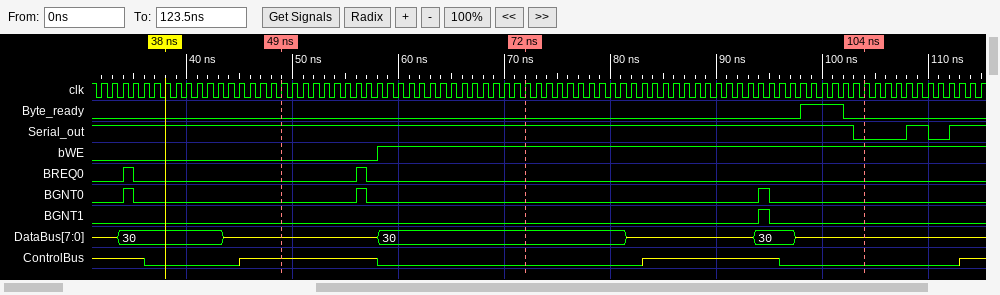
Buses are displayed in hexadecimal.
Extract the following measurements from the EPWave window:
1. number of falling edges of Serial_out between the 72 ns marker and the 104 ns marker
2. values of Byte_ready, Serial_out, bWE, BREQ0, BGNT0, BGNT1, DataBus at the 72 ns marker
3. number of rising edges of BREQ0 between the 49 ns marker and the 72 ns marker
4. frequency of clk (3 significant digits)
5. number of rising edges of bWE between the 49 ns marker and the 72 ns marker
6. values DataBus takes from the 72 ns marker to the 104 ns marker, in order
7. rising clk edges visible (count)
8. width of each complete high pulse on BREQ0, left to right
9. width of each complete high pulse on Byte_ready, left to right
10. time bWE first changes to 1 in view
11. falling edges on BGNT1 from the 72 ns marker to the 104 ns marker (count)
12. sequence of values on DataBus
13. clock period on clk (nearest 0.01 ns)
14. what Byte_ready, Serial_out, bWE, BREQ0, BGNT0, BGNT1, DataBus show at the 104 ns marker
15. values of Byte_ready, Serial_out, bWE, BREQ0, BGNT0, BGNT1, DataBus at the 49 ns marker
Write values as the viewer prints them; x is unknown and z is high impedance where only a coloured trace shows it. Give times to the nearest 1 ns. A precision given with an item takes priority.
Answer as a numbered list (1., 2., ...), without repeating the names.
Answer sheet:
1. 1
2. Byte_ready=0, Serial_out=1, bWE=1, BREQ0=0, BGNT0=0, BGNT1=0, DataBus=30
3. 1
4. 1.00 GHz
5. 1
6. 30, z, 30, z
7. 84
8. 1 ns, 1 ns
9. 4 ns
10. 58 ns
11. 1
12. z, 30, z, 30, z, 30, z
13. 1 ns
14. Byte_ready=0, Serial_out=0, bWE=1, BREQ0=0, BGNT0=0, BGNT1=0, DataBus=z
15. Byte_ready=0, Serial_out=1, bWE=0, BREQ0=0, BGNT0=0, BGNT1=0, DataBus=z
